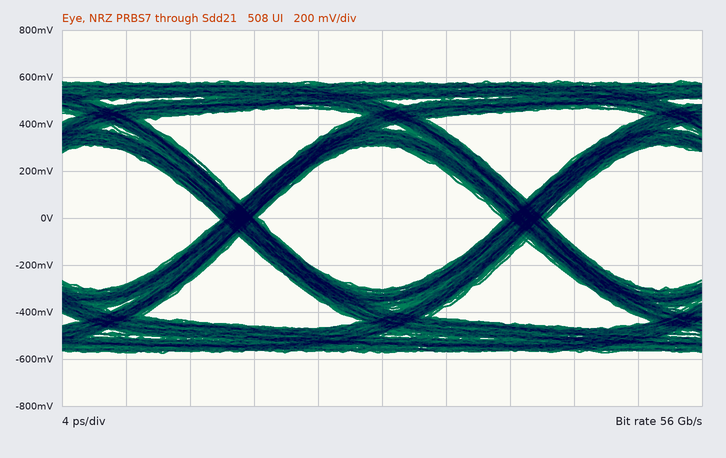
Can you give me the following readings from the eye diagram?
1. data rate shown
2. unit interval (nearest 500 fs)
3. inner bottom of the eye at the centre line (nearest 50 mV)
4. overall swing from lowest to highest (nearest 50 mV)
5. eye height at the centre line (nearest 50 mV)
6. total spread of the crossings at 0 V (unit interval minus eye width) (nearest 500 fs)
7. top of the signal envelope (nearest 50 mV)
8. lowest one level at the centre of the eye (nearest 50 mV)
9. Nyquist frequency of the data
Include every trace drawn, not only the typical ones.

56 Gb/s
18.0 ps
-300 mV
1.15 V
600 mV
2.5 ps
600 mV
300 mV
28 GHz
